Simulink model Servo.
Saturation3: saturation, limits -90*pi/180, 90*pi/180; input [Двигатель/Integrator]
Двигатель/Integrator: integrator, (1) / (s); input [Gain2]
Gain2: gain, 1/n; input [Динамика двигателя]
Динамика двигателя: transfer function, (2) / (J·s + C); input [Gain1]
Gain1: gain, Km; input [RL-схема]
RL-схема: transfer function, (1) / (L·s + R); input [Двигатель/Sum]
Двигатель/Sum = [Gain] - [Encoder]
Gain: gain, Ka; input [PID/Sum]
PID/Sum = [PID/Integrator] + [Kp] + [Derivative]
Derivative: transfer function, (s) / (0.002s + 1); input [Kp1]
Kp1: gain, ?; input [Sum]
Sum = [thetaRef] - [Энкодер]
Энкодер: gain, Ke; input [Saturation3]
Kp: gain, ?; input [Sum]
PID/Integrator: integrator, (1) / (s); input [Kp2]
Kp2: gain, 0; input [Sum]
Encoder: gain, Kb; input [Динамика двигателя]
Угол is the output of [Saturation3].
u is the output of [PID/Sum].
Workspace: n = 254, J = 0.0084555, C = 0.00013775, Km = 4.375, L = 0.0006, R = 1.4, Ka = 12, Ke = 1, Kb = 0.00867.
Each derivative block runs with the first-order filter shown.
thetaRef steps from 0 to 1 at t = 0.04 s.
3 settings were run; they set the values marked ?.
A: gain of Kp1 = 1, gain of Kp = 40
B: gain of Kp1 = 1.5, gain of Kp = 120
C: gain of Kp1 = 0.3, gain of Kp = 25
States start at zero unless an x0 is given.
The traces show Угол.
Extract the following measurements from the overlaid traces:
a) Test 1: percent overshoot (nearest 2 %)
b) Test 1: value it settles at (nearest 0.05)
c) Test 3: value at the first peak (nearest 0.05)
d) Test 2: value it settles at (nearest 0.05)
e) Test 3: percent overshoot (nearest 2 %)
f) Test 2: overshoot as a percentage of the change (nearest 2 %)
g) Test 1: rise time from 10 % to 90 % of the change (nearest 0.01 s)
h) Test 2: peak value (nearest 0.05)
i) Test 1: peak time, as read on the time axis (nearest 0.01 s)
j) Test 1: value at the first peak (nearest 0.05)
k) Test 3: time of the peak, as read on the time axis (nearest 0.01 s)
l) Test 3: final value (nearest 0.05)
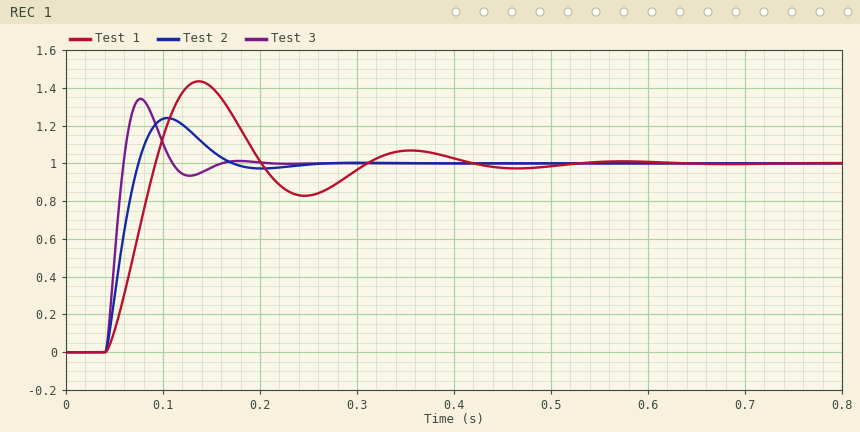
44 %
1.00
1.35
1.00
34 %
24 %
0.04 s
1.25
0.14 s
1.45
0.08 s
1.00
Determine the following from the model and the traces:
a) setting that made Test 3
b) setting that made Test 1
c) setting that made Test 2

B
C
A
